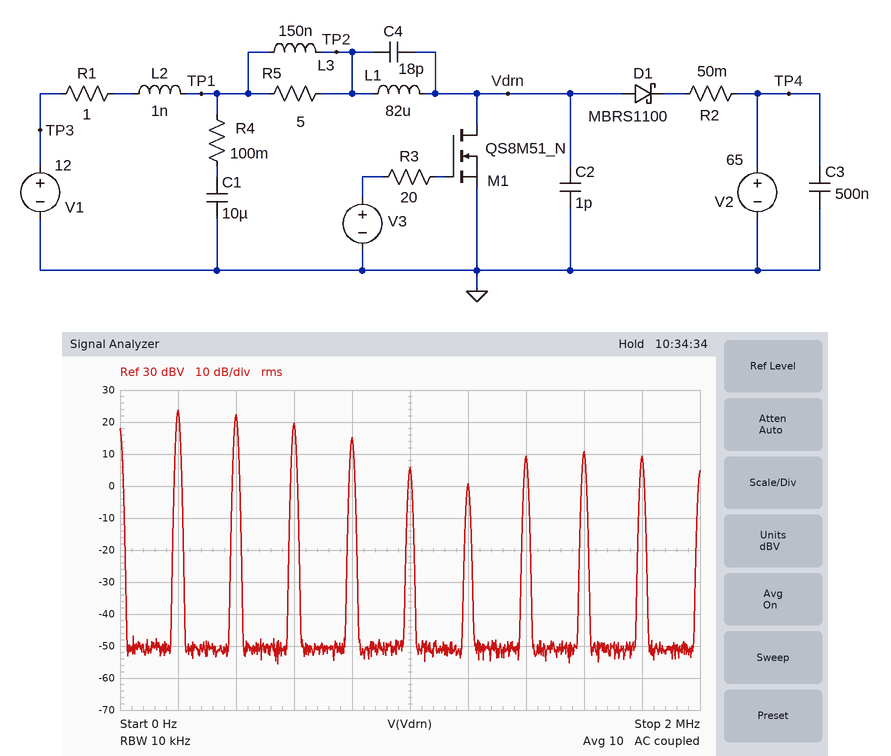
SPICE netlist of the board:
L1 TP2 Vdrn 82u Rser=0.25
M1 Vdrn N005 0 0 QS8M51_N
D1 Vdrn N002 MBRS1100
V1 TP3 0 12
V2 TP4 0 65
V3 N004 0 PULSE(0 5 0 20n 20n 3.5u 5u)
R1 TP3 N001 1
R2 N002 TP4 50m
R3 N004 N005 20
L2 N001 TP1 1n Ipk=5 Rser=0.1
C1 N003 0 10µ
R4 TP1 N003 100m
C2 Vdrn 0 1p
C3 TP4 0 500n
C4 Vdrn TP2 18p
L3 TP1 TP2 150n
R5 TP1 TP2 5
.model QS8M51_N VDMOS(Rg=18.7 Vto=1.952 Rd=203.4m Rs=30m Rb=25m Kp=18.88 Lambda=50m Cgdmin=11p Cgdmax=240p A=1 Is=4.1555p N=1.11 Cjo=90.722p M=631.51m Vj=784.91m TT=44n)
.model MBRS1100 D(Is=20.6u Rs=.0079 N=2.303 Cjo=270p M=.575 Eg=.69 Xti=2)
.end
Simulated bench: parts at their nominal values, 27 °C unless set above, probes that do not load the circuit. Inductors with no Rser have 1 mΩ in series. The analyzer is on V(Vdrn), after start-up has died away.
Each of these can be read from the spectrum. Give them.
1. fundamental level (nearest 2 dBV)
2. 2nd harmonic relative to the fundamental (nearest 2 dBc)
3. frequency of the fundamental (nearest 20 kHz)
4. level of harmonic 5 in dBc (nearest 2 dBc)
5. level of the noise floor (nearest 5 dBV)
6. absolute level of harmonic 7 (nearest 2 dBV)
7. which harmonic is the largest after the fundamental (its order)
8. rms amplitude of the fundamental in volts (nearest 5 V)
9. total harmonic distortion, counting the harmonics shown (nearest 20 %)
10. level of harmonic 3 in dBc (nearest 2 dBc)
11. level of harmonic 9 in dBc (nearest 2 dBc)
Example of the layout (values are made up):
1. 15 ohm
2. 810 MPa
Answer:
1. 24 dBV
2. -2 dBc
3. 200 kHz
4. -18 dBc
5. -50 dBV
6. 10 dBV
7. 2
8. 15 V
9. 120 %
10. -4 dBc
11. -14 dBc
